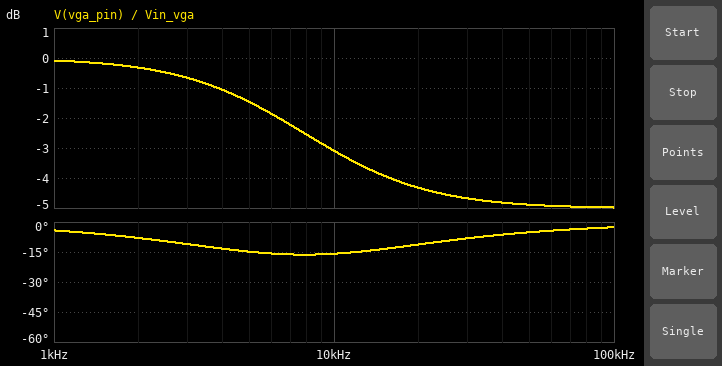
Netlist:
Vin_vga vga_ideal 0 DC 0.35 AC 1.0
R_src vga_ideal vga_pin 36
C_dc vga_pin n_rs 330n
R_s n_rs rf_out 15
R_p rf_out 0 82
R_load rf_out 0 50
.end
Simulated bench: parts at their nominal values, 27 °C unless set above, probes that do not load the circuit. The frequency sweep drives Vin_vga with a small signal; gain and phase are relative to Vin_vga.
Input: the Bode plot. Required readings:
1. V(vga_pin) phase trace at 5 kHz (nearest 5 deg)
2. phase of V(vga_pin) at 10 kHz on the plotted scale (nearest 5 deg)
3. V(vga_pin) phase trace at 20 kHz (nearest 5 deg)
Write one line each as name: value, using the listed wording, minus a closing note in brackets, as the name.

V(vga_pin) phase trace at 5 kHz: -15 deg
phase of V(vga_pin) at 10 kHz on the plotted scale: -15 deg
V(vga_pin) phase trace at 20 kHz: -10 deg
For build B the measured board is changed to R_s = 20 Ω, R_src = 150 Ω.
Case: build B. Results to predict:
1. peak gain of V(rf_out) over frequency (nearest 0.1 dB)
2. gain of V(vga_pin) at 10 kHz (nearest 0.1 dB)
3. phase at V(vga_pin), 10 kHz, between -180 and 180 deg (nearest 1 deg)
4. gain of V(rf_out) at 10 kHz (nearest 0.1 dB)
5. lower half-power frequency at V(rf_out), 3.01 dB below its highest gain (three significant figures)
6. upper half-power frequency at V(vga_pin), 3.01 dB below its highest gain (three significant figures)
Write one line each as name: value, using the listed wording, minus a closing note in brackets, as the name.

peak gain of V(rf_out) over frequency: -16.2 dB
gain of V(vga_pin) at 10 kHz: -9.4 dB
phase at V(vga_pin), 10 kHz, between -180 and 180 deg: -30 deg
gain of V(rf_out) at 10 kHz: -16.5 dB
lower half-power frequency at V(rf_out), 3.01 dB below its highest gain: 2.40 kHz
upper half-power frequency at V(vga_pin), 3.01 dB below its highest gain: 2.57 kHz
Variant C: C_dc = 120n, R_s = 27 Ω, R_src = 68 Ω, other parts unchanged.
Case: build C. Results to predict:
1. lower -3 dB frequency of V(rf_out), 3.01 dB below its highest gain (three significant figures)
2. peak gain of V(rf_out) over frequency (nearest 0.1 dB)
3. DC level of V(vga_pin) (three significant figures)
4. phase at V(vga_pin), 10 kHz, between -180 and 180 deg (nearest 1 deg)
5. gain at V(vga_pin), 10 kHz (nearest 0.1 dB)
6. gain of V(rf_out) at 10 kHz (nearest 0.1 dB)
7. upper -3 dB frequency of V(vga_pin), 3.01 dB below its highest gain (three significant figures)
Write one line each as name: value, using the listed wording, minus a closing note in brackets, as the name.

lower -3 dB frequency of V(rf_out), 3.01 dB below its highest gain: 10.5 kHz
peak gain of V(rf_out) over frequency: -12.2 dB
DC level of V(vga_pin): 350 mV
phase at V(vga_pin), 10 kHz, between -180 and 180 deg: -20 deg
gain at V(vga_pin), 10 kHz: -2.0 dB
gain of V(rf_out) at 10 kHz: -15.4 dB
upper -3 dB frequency of V(vga_pin), 3.01 dB below its highest gain: 13.9 kHz
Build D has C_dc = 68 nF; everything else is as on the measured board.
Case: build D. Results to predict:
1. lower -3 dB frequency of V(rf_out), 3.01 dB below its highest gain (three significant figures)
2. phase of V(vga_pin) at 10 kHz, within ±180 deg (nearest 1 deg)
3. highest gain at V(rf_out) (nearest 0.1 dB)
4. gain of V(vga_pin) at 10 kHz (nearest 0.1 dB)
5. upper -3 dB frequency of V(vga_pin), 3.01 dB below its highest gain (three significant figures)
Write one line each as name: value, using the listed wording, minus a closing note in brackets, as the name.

lower -3 dB frequency of V(rf_out), 3.01 dB below its highest gain: 28.5 kHz
phase of V(vga_pin) at 10 kHz, within ±180 deg: -8 deg
highest gain at V(rf_out): -8.4 dB
gain of V(vga_pin) at 10 kHz: -0.3 dB
upper -3 dB frequency of V(vga_pin), 3.01 dB below its highest gain: 46.9 kHz
